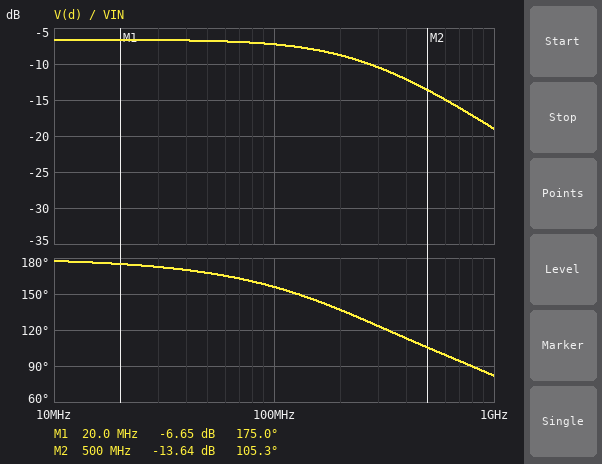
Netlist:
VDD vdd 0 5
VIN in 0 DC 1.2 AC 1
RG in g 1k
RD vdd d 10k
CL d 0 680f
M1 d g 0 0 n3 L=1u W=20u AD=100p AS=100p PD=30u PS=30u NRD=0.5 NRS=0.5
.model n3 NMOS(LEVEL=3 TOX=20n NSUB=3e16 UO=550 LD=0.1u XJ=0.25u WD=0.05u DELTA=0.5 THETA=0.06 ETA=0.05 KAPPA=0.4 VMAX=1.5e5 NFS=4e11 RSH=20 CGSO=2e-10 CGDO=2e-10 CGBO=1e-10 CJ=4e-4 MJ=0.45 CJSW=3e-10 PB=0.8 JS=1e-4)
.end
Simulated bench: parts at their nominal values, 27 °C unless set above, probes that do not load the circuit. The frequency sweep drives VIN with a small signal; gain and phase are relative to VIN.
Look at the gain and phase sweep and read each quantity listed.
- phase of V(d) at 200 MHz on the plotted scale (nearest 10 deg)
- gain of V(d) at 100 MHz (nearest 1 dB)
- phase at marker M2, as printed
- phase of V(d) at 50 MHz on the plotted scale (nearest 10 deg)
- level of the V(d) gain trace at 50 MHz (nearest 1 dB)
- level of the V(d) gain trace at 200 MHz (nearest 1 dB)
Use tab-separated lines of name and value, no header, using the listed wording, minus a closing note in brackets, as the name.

phase of V(d) at 200 MHz on the plotted scale	140 deg
gain of V(d) at 100 MHz	-7 dB
phase at marker M2, as printed	105.3 deg
phase of V(d) at 50 MHz on the plotted scale	170 deg
level of the V(d) gain trace at 50 MHz	-7 dB
level of the V(d) gain trace at 200 MHz	-9 dB
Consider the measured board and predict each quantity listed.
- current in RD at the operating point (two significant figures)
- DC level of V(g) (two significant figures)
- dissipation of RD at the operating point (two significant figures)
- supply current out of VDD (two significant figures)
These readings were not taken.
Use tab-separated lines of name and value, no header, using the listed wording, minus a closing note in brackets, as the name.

current in RD at the operating point	470 µA
DC level of V(g)	1.2 V
dissipation of RD at the operating point	2.2 mW
supply current out of VDD	470 µA
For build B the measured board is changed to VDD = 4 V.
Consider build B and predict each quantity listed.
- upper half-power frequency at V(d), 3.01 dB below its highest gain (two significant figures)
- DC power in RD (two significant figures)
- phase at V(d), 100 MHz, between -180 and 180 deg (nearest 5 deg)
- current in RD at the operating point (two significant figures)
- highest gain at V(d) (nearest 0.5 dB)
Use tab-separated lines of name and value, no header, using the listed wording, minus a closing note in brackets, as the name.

upper half-power frequency at V(d), 3.01 dB below its highest gain	300 MHz
DC power in RD	1.4 mW
phase at V(d), 100 MHz, between -180 and 180 deg	160 deg
current in RD at the operating point	380 µA
highest gain at V(d)	-10.5 dB
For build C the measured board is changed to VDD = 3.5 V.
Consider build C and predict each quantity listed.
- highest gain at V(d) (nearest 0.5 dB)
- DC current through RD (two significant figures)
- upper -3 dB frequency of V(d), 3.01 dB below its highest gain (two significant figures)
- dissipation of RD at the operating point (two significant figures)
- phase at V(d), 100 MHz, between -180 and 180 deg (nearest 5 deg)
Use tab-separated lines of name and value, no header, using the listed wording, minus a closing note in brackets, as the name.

highest gain at V(d)	-12.5 dB
DC current through RD	330 µA
upper -3 dB frequency of V(d), 3.01 dB below its highest gain	320 MHz
dissipation of RD at the operating point	1.1 mW
phase at V(d), 100 MHz, between -180 and 180 deg	160 deg
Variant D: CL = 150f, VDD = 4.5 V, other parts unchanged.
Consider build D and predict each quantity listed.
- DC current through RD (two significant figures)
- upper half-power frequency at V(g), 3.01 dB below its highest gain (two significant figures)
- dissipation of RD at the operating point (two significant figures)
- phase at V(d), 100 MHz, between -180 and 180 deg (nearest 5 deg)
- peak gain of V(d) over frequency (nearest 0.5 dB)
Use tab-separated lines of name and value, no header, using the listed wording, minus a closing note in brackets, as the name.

DC current through RD	420 µA
upper half-power frequency at V(g), 3.01 dB below its highest gain	4.4 GHz
dissipation of RD at the operating point	1.8 mW
phase at V(d), 100 MHz, between -180 and 180 deg	170 deg
peak gain of V(d) over frequency	-8.5 dB
